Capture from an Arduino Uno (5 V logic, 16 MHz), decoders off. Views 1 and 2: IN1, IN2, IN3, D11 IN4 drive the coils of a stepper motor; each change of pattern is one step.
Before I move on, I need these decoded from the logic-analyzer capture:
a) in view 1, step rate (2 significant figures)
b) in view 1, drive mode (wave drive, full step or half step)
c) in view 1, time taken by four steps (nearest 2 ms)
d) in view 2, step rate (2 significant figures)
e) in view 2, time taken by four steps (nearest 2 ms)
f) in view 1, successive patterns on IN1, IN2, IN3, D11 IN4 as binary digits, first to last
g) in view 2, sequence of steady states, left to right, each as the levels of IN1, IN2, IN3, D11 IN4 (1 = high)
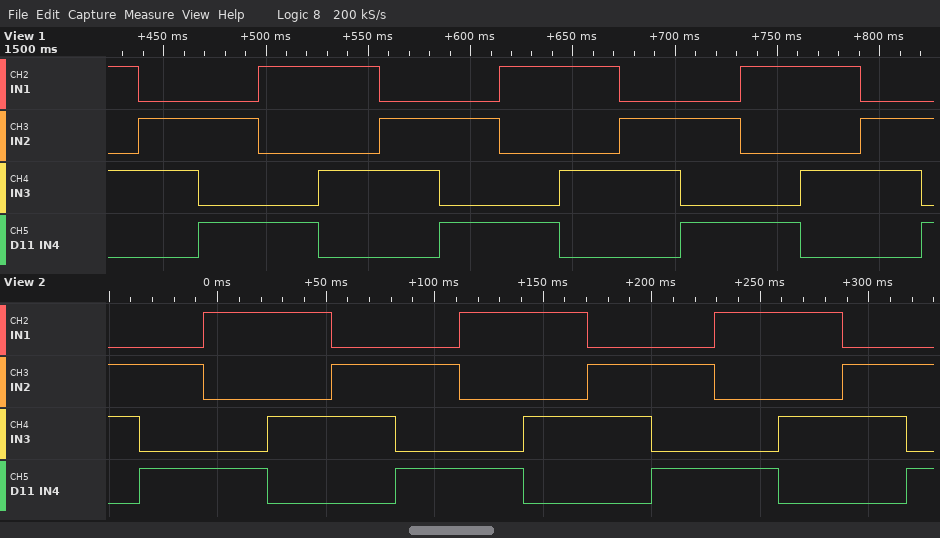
34 steps/s
full step
118 ms
34 steps/s
118 ms
1010 0110 0101 1001 1010 0110 0101 1001 1010 0110 0101 1001 1010 0110 0101
0110 0101 1001 1010 0110 0101 1001 1010 0110 0101 1001 1010 0110 0101
